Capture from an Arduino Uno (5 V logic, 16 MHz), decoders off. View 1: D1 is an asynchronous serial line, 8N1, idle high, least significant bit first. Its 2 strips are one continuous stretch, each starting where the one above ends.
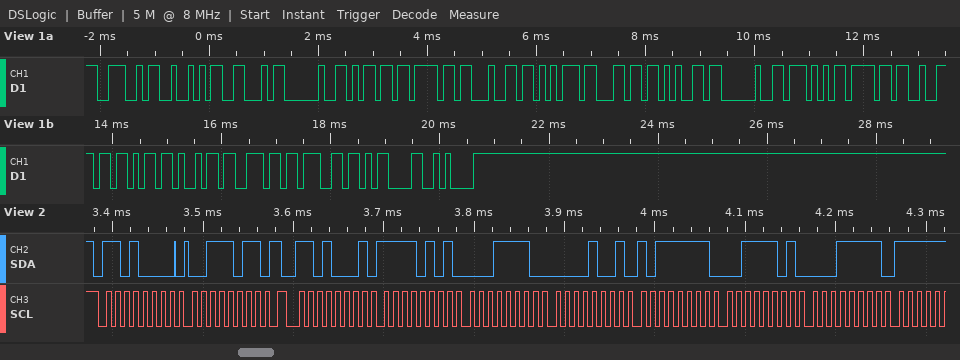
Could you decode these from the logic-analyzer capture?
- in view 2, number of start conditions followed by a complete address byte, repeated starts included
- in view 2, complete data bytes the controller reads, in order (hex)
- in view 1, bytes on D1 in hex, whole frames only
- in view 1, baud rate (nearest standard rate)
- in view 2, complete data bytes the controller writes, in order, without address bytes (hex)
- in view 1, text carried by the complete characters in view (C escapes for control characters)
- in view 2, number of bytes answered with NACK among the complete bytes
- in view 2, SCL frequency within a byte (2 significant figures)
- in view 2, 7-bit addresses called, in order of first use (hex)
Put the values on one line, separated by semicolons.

2; F5 1E 09 BF 3D 1F; 0x4E 0x52 0x46 0x20 0x6D 0x6F 0x64 0x75 0x6C 0x65 0x20 0x57 0x6F 0x72 0x6B 0x69 0x6E 0x67 0x0D 0x0A; 9600 baud; 3B; "NRF module Working\r\n"; 0; 100 kHz; 0x68
